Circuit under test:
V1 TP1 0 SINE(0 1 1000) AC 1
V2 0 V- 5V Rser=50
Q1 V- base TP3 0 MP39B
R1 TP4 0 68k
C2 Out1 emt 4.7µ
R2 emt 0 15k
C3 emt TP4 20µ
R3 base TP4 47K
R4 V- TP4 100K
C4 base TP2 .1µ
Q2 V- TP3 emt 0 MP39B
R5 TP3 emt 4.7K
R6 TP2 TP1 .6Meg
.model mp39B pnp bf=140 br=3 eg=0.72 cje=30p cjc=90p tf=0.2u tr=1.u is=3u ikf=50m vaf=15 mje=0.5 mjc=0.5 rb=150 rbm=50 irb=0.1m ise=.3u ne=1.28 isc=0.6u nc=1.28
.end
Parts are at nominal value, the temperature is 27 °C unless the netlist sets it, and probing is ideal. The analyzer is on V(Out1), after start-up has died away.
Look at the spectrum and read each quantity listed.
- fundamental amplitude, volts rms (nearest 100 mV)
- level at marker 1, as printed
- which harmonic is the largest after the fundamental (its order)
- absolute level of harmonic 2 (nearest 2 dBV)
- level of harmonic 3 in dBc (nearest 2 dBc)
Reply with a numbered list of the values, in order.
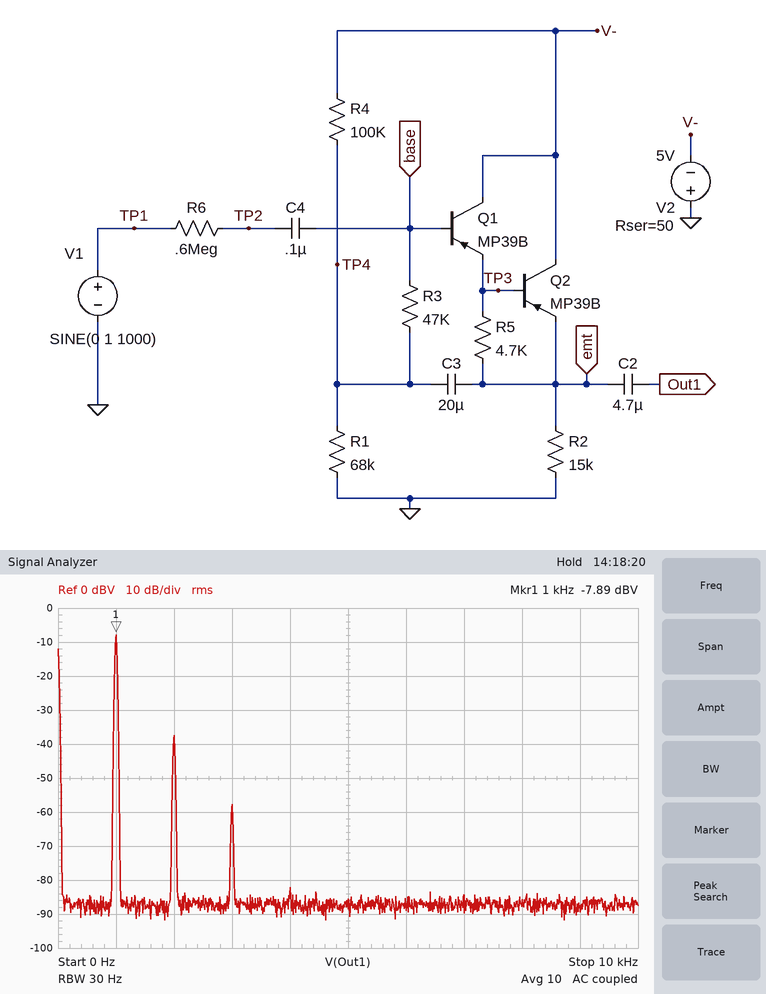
1. 400 mV
2. -7.89 dBV
3. 2
4. -38 dBV
5. -50 dBc
